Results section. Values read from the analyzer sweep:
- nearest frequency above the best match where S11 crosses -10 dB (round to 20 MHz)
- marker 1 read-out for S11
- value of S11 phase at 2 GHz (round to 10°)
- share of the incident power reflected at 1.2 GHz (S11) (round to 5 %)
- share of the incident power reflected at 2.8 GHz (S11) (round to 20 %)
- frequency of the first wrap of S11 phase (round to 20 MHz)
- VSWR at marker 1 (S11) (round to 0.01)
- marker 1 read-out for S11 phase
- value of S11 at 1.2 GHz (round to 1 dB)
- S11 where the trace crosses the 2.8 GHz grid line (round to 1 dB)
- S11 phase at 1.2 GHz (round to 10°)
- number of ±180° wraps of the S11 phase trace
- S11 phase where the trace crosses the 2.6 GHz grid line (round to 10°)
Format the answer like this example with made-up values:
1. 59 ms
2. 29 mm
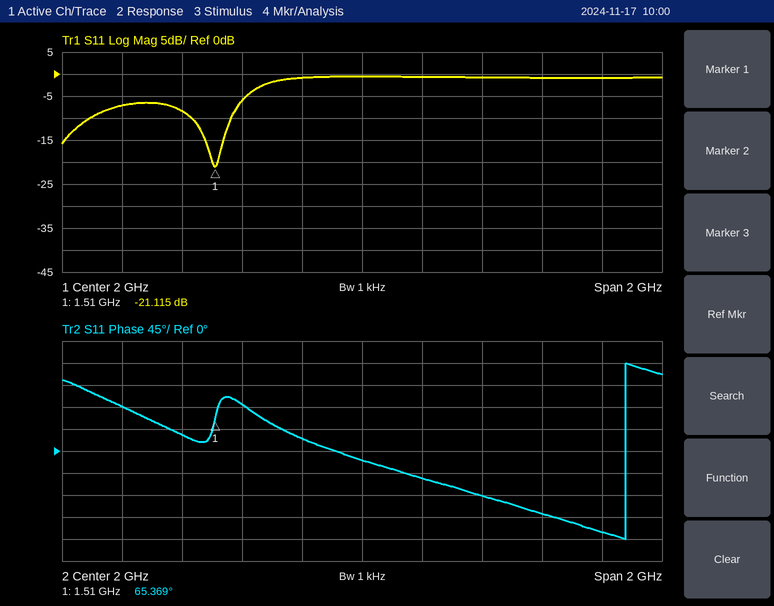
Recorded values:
1. 1.56 GHz
2. -21.115 dB
3. -20°
4. 20 %
5. 80 %
6. 2.88 GHz
7. 1.19
8. 65.369°
9. -7 dB
10. -1 dB
11. 90°
12. 1
13. -130°
